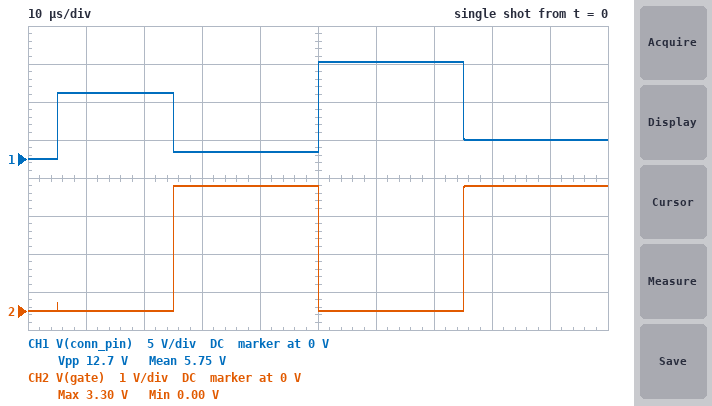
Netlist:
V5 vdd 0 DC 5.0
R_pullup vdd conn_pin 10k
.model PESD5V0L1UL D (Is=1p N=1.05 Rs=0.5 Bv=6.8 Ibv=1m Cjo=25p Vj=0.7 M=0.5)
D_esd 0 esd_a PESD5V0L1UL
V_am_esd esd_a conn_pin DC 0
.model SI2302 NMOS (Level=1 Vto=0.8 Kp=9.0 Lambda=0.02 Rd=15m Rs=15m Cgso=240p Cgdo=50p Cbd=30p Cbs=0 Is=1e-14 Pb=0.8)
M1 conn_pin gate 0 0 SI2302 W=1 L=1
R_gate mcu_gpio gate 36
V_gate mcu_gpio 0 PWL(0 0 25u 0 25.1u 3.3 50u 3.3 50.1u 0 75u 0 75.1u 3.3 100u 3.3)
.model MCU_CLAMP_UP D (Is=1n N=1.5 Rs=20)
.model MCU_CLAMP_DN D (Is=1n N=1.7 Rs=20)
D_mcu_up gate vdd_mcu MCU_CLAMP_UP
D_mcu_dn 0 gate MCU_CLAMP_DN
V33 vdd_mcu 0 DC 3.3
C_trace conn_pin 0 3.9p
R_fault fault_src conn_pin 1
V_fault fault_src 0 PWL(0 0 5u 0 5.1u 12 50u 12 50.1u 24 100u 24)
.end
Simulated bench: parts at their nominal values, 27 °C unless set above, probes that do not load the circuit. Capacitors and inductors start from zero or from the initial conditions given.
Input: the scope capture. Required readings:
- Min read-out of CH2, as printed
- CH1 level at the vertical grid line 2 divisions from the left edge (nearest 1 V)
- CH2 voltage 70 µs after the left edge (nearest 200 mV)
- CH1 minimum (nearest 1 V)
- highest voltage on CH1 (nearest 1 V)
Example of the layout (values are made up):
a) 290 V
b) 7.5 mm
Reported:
a) 0.00 V
b) 9 V
c) 0 V
d) 0 V
e) 13 V
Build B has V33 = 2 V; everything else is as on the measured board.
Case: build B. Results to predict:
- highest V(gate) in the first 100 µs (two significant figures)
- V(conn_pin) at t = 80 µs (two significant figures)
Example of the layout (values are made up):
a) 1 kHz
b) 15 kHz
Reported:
a) 2.9 V
b) 7.0 V
